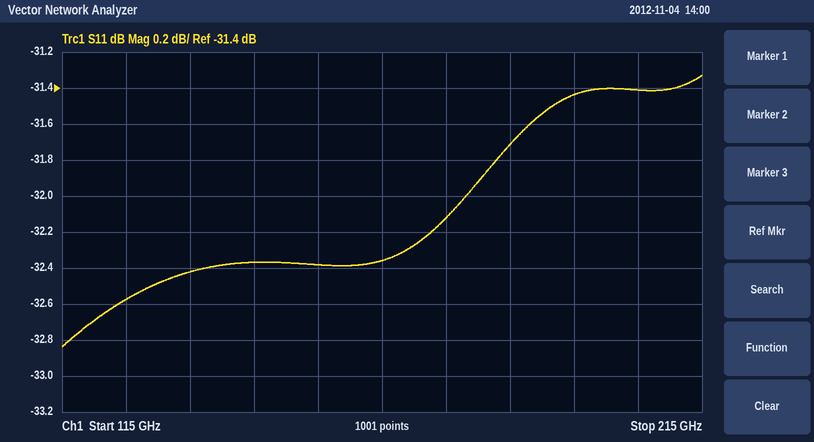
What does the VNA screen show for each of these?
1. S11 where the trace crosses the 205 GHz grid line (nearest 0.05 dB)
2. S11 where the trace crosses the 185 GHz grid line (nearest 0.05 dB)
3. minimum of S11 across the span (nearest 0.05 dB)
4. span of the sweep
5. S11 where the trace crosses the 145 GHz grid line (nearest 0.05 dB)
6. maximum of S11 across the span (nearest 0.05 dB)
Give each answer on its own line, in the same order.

-31.40 dB
-31.70 dB
-32.85 dB
100 GHz
-32.35 dB
-31.35 dB
